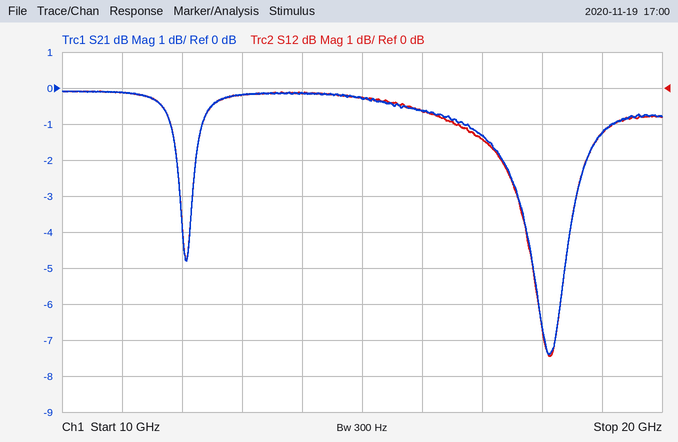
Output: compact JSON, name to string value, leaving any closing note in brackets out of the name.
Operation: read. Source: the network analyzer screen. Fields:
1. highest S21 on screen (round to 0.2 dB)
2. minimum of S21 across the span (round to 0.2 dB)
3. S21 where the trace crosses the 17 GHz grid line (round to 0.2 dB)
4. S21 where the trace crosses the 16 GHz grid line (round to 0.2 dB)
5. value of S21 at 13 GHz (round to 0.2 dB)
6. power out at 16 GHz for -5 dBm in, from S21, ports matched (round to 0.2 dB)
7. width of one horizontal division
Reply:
{"highest S21 on screen": "0.0 dB", "minimum of S21 across the span": "-7.4 dB", "S21 where the trace crosses the 17 GHz grid line": "-1.4 dB", "S21 where the trace crosses the 16 GHz grid line": "-0.6 dB", "value of S21 at 13 GHz": "-0.2 dB", "power out at 16 GHz for -5 dBm in, from S21, ports matched": "-5.6 dBm", "width of one horizontal division": "1 GHz"}
